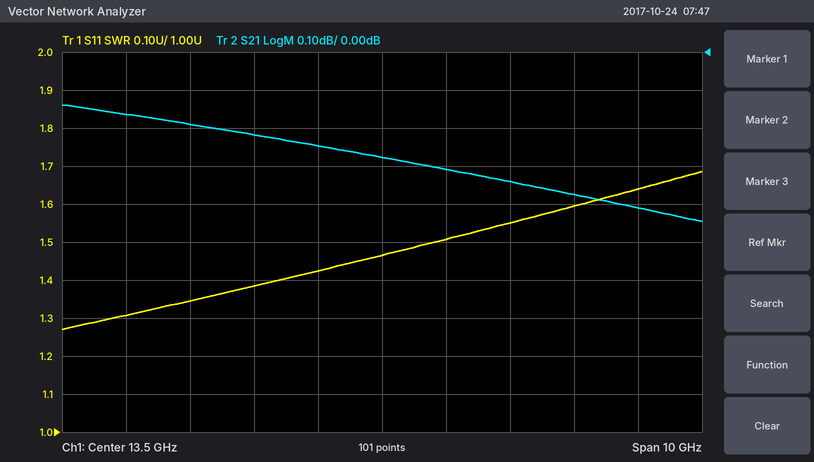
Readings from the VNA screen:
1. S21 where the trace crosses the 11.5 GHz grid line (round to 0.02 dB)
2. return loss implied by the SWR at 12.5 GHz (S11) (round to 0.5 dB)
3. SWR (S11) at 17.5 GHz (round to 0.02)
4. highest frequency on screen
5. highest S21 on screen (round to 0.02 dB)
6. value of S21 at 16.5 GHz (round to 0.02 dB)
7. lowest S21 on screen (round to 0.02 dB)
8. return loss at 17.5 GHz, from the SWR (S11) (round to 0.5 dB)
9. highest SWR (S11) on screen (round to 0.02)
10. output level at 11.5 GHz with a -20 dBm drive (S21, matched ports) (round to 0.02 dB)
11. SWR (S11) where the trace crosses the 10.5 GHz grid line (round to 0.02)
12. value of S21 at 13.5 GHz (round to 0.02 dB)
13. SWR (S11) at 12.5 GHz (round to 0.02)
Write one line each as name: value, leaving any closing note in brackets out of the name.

S21 where the trace crosses the 11.5 GHz grid line: -0.22 dB
return loss implied by the SWR at 12.5 GHz (S11): 15.0 dB
SWR (S11) at 17.5 GHz: 1.64
highest frequency on screen: 18.5 GHz
highest S21 on screen: -0.14 dB
value of S21 at 16.5 GHz: -0.38 dB
lowest S21 on screen: -0.44 dB
return loss at 17.5 GHz, from the SWR (S11): 12.5 dB
highest SWR (S11) on screen: 1.68
output level at 11.5 GHz with a -20 dBm drive (S21, matched ports): -20.22 dBm
SWR (S11) where the trace crosses the 10.5 GHz grid line: 1.34
value of S21 at 13.5 GHz: -0.28 dB
SWR (S11) at 12.5 GHz: 1.42
